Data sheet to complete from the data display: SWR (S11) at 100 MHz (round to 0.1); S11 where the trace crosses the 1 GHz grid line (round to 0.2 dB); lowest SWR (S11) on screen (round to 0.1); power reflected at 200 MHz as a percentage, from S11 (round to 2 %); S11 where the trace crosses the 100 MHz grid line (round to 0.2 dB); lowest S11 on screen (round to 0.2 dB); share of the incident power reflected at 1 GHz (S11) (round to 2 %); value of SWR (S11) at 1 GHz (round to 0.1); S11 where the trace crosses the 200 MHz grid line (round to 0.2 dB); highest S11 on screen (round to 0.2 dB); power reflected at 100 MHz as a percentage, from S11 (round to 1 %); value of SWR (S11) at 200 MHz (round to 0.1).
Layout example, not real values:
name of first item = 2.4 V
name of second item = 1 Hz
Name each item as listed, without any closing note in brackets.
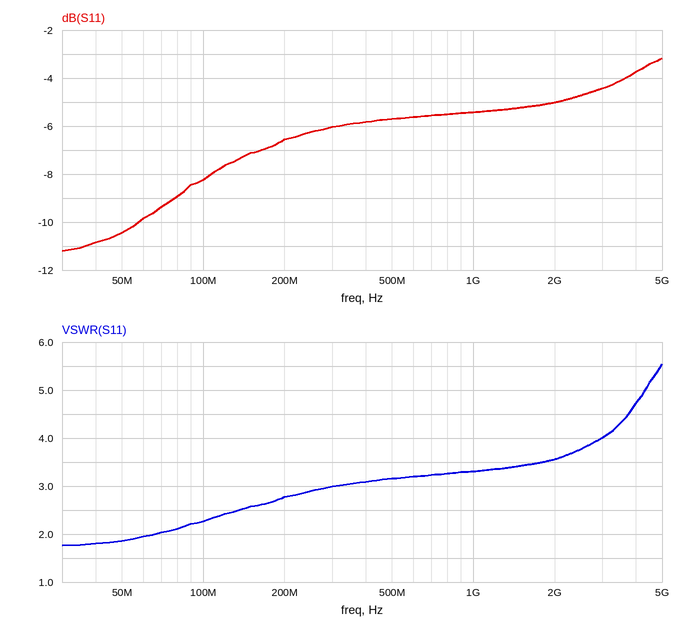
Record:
SWR (S11) at 100 MHz = 2.3
S11 where the trace crosses the 1 GHz grid line = -5.4 dB
lowest SWR (S11) on screen = 1.8
power reflected at 200 MHz as a percentage, from S11 = 22 %
S11 where the trace crosses the 100 MHz grid line = -8.2 dB
lowest S11 on screen = -11.2 dB
share of the incident power reflected at 1 GHz (S11) = 28 %
value of SWR (S11) at 1 GHz = 3.3
S11 where the trace crosses the 200 MHz grid line = -6.6 dB
highest S11 on screen = -3.2 dB
power reflected at 100 MHz as a percentage, from S11 = 15 %
value of SWR (S11) at 200 MHz = 2.8
